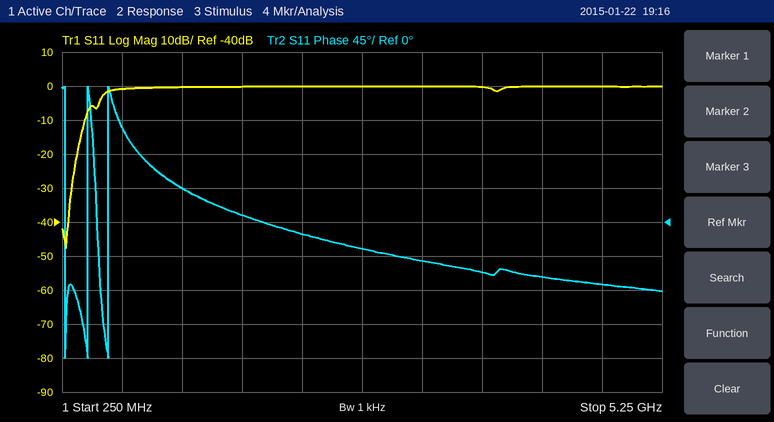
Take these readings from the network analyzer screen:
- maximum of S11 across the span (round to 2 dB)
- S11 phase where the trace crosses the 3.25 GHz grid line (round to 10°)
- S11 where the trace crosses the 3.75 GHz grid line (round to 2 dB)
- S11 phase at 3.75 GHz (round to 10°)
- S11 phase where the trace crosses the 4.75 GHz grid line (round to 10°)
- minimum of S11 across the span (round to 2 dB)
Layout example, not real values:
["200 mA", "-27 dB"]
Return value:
["0 dB", "-50°", "0 dB", "-70°", "-80°", "-48 dB"]
